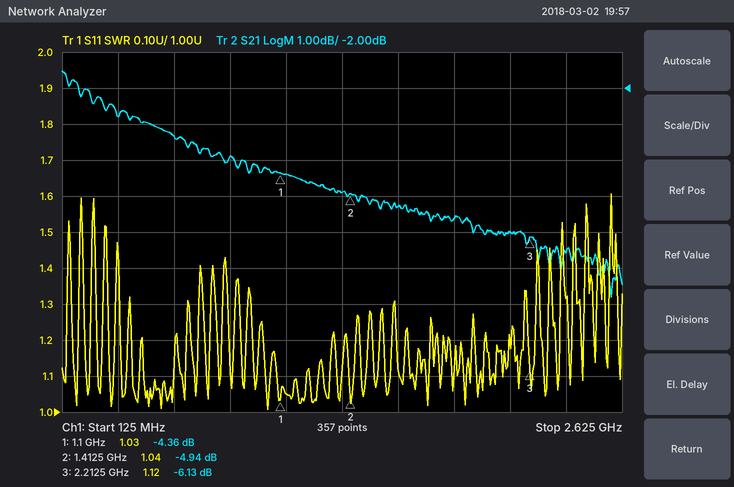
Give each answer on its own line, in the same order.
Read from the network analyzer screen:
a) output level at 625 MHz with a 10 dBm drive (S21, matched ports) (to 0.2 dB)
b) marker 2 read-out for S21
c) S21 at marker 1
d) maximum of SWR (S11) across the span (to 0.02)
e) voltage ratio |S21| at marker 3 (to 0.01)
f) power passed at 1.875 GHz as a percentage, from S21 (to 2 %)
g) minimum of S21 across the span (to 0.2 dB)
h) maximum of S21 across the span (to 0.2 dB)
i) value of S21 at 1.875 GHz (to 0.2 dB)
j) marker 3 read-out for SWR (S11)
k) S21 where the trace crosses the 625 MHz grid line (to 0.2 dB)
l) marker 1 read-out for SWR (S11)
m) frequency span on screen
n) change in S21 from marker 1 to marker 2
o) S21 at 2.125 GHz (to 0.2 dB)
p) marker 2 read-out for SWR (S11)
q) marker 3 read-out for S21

6.6 dBm
-4.94 dB
-4.36 dB
1.60
0.49
28 %
-7.8 dB
-1.6 dB
-5.6 dB
1.12
-3.4 dB
1.03
2.5 GHz
-0.58 dB
-6.0 dB
1.04
-6.13 dB
